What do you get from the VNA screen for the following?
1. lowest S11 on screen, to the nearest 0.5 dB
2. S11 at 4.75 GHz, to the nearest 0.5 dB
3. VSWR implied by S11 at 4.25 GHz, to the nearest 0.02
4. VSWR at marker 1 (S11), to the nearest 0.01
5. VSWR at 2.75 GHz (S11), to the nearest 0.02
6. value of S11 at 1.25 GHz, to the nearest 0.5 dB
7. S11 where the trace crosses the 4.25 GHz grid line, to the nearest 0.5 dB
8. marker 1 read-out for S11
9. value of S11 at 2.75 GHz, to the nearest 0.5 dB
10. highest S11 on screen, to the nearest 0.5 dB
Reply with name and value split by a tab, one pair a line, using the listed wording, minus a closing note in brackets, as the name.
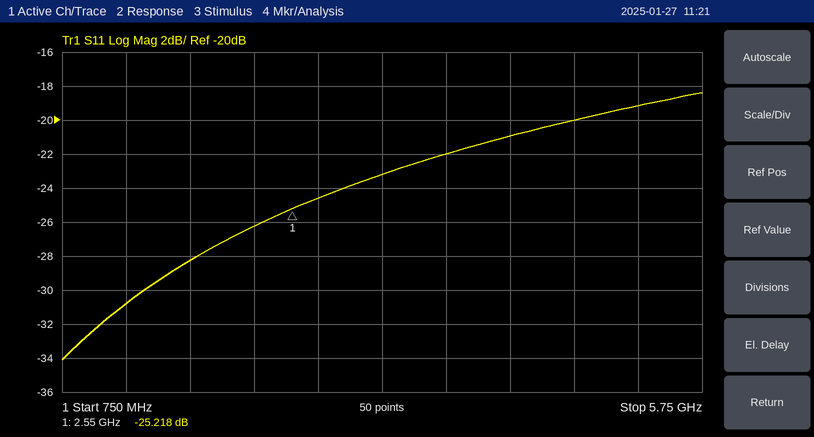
lowest S11 on screen, to the nearest 0.5 dB	-34.0 dB
S11 at 4.75 GHz, to the nearest 0.5 dB	-20.0 dB
VSWR implied by S11 at 4.25 GHz, to the nearest 0.02	1.20
VSWR at marker 1 (S11), to the nearest 0.01	1.12
VSWR at 2.75 GHz (S11), to the nearest 0.02	1.12
value of S11 at 1.25 GHz, to the nearest 0.5 dB	-31.0 dB
S11 where the trace crosses the 4.25 GHz grid line, to the nearest 0.5 dB	-21.0 dB
marker 1 read-out for S11	-25.218 dB
value of S11 at 2.75 GHz, to the nearest 0.5 dB	-24.5 dB
highest S11 on screen, to the nearest 0.5 dB	-18.5 dB
